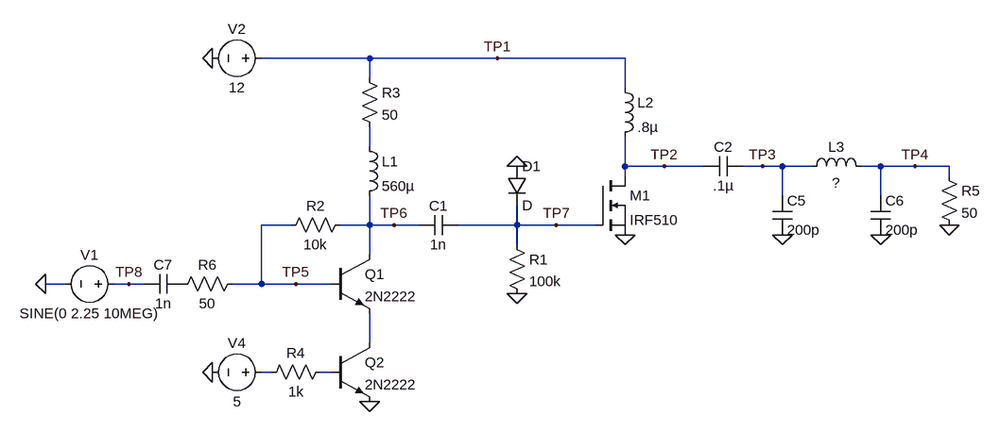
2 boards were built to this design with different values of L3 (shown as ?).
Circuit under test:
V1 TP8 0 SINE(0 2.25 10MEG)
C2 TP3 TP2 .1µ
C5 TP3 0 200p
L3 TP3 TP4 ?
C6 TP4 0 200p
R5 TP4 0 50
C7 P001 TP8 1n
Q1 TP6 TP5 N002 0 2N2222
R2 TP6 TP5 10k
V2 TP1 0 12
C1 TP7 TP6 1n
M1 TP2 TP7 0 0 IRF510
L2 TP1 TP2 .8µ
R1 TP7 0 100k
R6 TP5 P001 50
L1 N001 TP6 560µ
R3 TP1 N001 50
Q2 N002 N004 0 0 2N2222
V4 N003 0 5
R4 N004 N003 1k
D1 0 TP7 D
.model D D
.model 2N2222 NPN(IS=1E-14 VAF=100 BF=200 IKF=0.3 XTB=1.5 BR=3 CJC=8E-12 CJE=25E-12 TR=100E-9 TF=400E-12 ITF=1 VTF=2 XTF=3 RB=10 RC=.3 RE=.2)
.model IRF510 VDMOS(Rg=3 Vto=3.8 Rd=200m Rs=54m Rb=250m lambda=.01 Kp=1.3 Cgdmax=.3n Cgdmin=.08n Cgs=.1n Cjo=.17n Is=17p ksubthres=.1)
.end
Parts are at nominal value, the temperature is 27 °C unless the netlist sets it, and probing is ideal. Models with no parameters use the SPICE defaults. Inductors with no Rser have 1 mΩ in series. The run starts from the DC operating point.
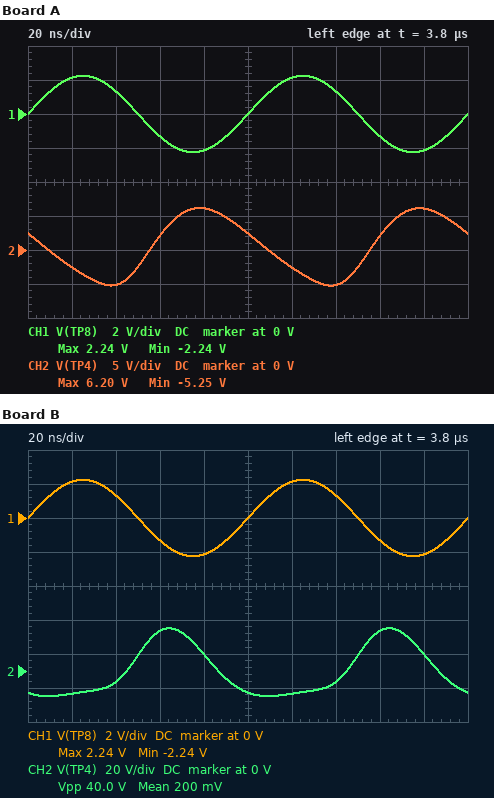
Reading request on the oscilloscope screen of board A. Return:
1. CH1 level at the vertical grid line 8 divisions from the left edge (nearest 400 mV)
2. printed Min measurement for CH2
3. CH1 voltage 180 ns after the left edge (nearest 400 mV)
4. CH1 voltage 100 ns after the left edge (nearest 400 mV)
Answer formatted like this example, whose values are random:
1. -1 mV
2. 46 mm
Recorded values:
1. -1.2 V
2. -5.25 V
3. -2.0 V
4. 0 V
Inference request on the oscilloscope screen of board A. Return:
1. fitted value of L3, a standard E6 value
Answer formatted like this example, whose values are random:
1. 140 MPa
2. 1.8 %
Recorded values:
1. 2.2 µH
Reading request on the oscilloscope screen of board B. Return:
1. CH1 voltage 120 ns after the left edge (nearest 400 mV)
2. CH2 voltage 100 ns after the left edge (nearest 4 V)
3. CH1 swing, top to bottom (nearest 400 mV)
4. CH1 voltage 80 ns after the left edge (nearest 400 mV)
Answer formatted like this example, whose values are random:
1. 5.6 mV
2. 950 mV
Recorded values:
1. 2.0 V
2. -12 V
3. 4.4 V
4. -2.0 V
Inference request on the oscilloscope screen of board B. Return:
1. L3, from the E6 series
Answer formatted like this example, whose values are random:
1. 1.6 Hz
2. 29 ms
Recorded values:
1. 470 nH
